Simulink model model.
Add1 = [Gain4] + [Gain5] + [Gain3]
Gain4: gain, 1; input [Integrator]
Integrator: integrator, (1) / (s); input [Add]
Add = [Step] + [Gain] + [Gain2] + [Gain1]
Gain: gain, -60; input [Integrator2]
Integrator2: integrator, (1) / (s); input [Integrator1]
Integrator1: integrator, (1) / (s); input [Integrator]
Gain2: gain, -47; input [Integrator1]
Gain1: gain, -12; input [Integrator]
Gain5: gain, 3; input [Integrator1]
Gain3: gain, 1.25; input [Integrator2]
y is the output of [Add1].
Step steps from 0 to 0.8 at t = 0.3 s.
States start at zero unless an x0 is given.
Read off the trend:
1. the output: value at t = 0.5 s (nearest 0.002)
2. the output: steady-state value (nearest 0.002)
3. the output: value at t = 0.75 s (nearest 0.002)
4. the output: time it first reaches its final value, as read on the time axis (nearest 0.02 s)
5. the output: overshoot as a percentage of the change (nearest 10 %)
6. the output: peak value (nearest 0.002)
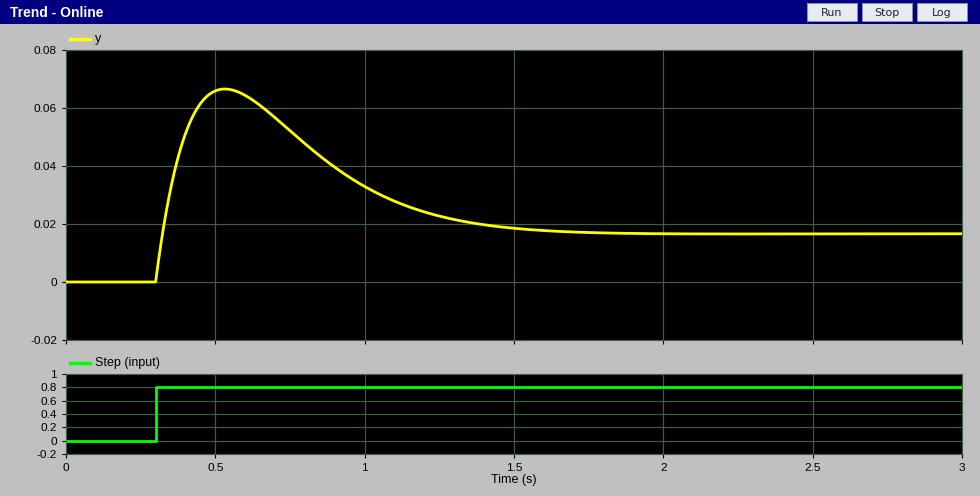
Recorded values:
0.066
0.016
0.052
0.32 s
300 %
0.066
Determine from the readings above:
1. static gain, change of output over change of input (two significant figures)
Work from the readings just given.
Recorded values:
0.020
